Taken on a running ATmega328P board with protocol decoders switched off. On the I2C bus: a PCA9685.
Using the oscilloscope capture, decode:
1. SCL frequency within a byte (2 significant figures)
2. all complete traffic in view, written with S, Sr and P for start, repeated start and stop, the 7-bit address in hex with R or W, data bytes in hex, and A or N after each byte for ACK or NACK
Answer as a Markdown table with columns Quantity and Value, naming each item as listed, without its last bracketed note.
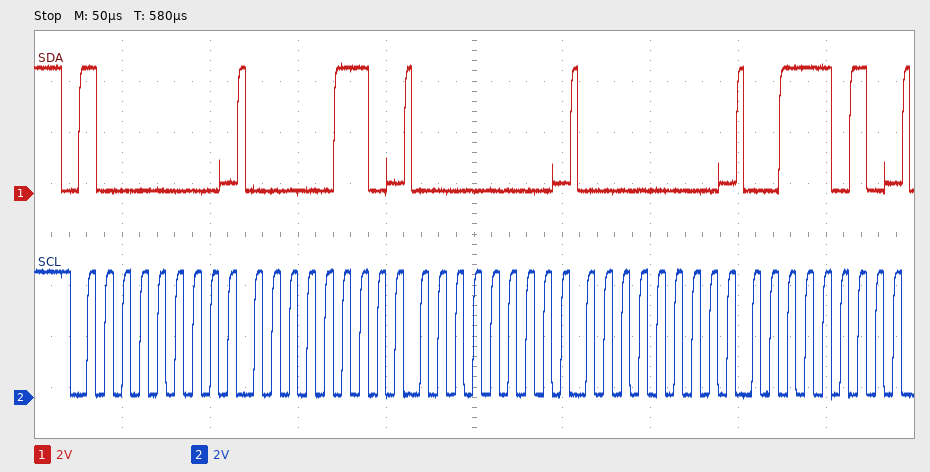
| Quantity | Value |
|---|---|
| SCL frequency within a byte | 100 kHz |
| all complete traffic in view, written with S, Sr and P for start, repeated start and stop, the 7-bit address in hex with R or W, data bytes in hex, and A or N after each byte for ACK or NACK | S 40W A 06 A 00 A 00 A 3A A |
